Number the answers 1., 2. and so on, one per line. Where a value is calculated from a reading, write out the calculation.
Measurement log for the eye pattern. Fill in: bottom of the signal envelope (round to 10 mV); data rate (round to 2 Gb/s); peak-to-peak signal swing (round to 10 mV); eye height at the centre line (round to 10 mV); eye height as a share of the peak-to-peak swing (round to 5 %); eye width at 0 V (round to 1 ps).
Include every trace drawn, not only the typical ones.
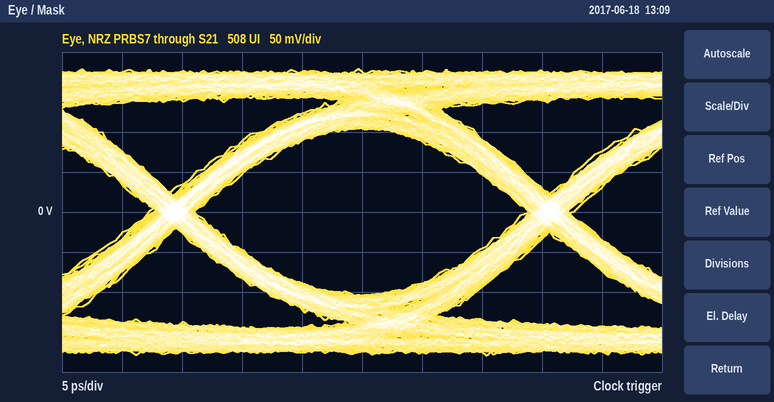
1. -180 mV
2. 32 Gb/s
3. 360 mV
4. 210 mV
5. 210 mV / 360 mV ≈ 58.3 %, so 60 % to the nearest 5 %
6. 28 ps
